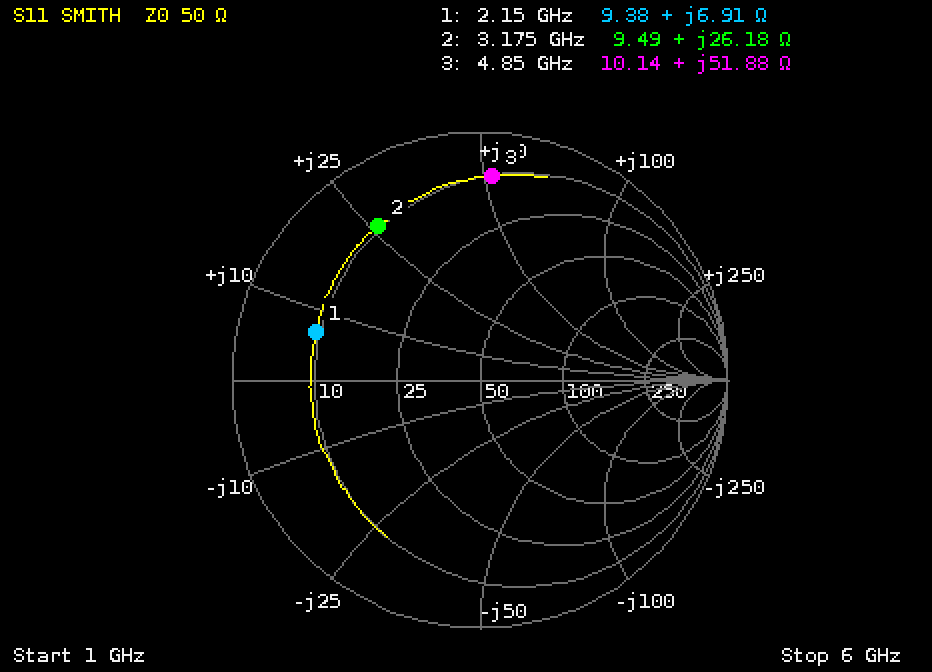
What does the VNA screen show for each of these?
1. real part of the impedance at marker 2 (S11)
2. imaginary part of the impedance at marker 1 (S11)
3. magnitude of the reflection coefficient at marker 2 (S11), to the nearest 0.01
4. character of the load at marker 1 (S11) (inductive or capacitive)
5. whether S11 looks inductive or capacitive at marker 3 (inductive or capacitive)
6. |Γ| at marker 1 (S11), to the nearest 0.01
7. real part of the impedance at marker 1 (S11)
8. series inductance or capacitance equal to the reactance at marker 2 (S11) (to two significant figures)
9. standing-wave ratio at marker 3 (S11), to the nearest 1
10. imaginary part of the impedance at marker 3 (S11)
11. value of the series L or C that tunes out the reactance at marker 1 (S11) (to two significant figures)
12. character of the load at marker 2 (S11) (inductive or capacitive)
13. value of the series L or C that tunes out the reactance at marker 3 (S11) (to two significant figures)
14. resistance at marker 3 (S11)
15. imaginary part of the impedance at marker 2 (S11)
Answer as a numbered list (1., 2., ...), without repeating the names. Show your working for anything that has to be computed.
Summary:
1. 9.49 Ω
2. +6.91 Ω
3. 0.74
4. inductive
5. inductive
6. 0.69
7. 9.38 Ω
8. L = 26.18 Ω/(2π × 3.175 GHz) ≈ 1.3 nH
9. 10
10. +51.88 Ω
11. C = 1/(2π × 2.15 GHz × 6.91 Ω) ≈ 11 pF
12. inductive
13. C = 1/(2π × 4.85 GHz × 51.88 Ω) ≈ 633 fF, so 630 fF to two significant figures
14. 10.14 Ω
15. +26.18 Ω
